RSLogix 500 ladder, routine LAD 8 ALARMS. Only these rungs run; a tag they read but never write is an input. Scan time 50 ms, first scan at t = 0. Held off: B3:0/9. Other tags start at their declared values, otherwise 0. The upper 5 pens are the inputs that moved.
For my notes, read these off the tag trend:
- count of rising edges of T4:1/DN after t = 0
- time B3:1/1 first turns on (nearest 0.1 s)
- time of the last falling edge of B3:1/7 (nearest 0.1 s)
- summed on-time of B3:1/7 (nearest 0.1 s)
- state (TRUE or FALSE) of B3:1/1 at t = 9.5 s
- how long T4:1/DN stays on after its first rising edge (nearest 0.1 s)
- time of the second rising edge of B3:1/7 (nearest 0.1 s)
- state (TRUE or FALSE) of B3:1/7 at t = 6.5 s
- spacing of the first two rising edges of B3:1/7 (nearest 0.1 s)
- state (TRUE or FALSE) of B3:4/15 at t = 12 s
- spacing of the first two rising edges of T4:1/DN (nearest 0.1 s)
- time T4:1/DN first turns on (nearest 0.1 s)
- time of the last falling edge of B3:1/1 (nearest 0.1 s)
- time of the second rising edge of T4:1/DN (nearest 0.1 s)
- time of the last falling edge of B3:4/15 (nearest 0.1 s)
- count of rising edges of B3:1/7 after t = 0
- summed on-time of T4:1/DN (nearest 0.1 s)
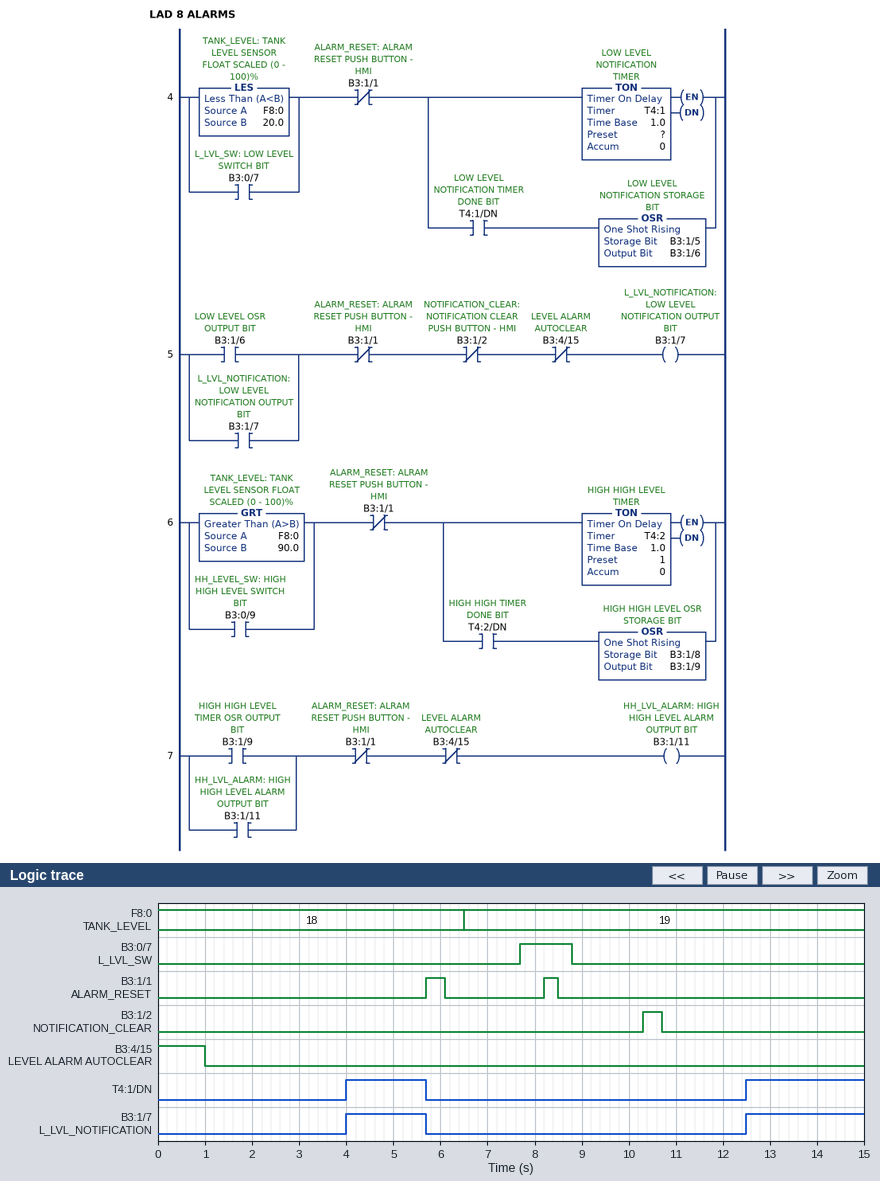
2
5.7 s
5.7 s
4.2 s
FALSE
1.7 s
12.5 s
FALSE
8.5 s
FALSE
8.5 s
4.0 s
8.5 s
12.5 s
1.0 s
2
4.2 s
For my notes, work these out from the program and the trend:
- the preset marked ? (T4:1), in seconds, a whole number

4 s
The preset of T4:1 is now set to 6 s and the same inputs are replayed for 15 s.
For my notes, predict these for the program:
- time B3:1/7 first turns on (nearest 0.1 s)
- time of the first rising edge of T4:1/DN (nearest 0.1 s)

14.5 s
14.5 s
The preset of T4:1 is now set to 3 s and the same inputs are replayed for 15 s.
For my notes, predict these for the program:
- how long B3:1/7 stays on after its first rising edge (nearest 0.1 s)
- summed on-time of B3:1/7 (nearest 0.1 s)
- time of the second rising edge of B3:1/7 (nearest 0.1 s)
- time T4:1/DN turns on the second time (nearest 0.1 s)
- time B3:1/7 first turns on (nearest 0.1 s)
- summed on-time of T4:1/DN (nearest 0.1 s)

2.7 s
6.2 s
11.5 s
11.5 s
3.0 s
6.2 s
